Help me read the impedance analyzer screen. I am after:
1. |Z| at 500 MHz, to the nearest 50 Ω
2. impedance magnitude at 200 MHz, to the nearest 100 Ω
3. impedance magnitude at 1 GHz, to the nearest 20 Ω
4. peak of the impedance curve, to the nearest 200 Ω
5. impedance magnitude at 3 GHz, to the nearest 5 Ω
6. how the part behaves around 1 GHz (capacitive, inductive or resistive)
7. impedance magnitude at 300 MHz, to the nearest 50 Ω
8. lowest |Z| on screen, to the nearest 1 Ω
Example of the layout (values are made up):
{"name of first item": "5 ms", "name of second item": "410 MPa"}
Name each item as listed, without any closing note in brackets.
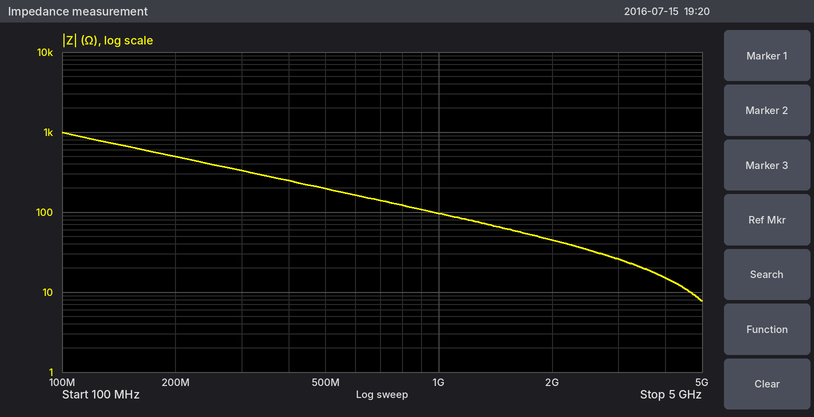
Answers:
{"|Z| at 500 MHz, to the nearest 50 Ω": "200 Ω", "impedance magnitude at 200 MHz, to the nearest 100 Ω": "500 Ω", "impedance magnitude at 1 GHz, to the nearest 20 Ω": "100 Ω", "peak of the impedance curve, to the nearest 200 Ω": "1.0 kΩ", "impedance magnitude at 3 GHz, to the nearest 5 Ω": "25 Ω", "how the part behaves around 1 GHz": "capacitive", "impedance magnitude at 300 MHz, to the nearest 50 Ω": "350 Ω", "lowest |Z| on screen, to the nearest 1 Ω": "8 Ω"}
